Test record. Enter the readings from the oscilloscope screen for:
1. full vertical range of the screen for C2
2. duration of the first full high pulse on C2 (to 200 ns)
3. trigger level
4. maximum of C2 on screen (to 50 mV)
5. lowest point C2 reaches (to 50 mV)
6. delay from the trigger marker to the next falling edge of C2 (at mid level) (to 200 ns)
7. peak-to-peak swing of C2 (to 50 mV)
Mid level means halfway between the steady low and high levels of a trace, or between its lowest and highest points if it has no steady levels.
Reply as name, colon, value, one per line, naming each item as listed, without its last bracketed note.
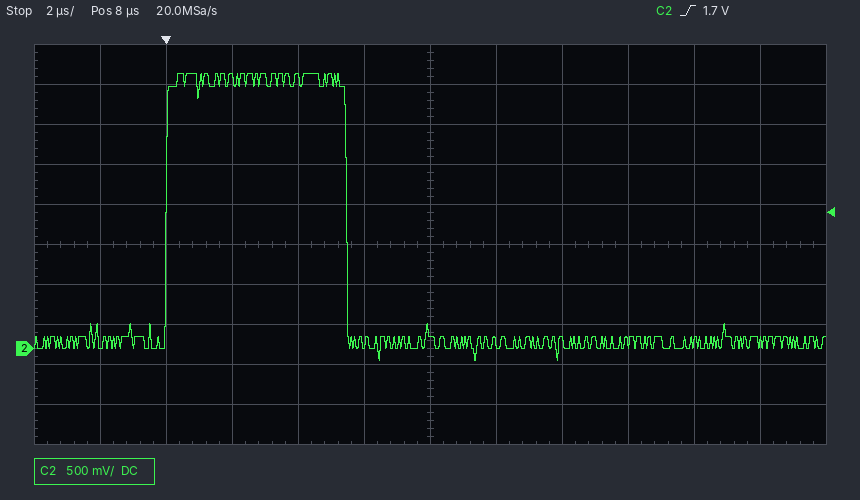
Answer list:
full vertical range of the screen for C2: 5 V
duration of the first full high pulse on C2: 5.4 µs
trigger level: 1.7 V
maximum of C2 on screen: 3.45 V
lowest point C2 reaches: -150 mV
delay from the trigger marker to the next falling edge of C2 (at mid level): 5.4 µs
peak-to-peak swing of C2: 3.60 V
